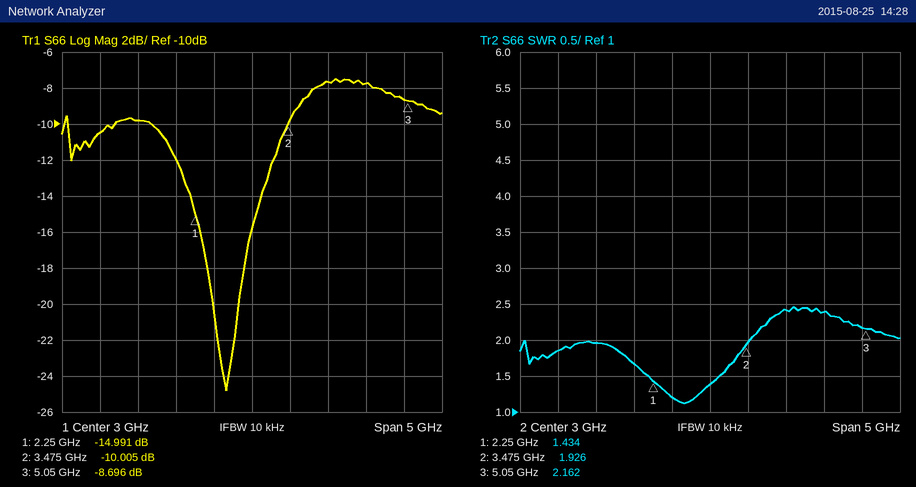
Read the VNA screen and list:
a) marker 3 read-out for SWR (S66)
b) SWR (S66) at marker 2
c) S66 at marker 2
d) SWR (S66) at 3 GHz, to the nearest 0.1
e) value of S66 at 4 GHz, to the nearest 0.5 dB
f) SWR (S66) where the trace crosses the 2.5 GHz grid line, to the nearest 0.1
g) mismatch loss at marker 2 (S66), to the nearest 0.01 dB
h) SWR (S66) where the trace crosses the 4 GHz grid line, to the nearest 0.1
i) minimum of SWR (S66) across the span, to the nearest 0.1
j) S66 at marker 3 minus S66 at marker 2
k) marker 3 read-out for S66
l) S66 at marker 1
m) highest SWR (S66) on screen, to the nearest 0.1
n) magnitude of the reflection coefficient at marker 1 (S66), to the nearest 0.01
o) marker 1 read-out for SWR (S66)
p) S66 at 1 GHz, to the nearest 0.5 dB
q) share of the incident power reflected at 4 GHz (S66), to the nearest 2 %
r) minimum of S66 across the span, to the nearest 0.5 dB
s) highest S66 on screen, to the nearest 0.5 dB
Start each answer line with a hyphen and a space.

- 2.162
- 1.926
- -10.005 dB
- 1.4
- -7.5 dB
- 1.2
- 0.46 dB
- 2.4
- 1.1
- 1.309 dB
- -8.696 dB
- -14.991 dB
- 2.5
- 0.18
- 1.434
- -10.5 dB
- 18 %
- -25.0 dB
- -7.5 dB
